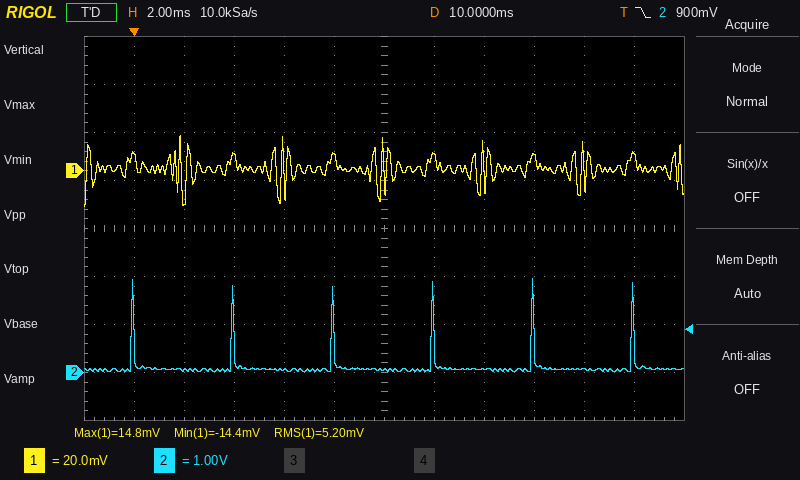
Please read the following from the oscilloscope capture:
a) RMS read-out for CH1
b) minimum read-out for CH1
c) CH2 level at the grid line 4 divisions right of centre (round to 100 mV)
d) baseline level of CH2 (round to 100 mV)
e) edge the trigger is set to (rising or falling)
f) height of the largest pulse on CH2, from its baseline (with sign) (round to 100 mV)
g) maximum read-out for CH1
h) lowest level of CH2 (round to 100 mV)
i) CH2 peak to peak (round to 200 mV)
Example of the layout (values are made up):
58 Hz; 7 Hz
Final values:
5.20 mV; -14.4 mV; 100 mV; 100 mV; falling; +1.9 V; 14.8 mV; 0.0 V; 2.0 V
